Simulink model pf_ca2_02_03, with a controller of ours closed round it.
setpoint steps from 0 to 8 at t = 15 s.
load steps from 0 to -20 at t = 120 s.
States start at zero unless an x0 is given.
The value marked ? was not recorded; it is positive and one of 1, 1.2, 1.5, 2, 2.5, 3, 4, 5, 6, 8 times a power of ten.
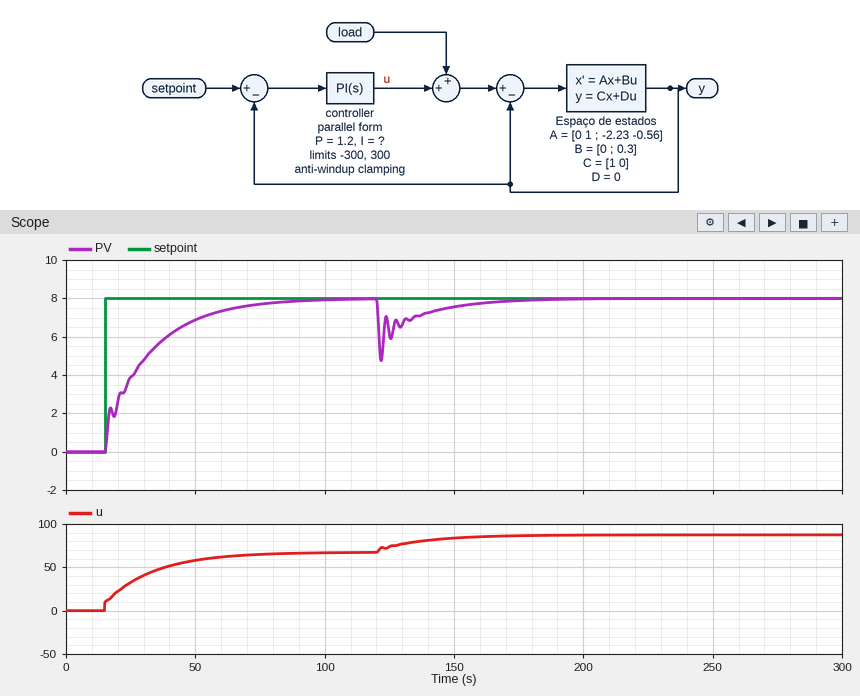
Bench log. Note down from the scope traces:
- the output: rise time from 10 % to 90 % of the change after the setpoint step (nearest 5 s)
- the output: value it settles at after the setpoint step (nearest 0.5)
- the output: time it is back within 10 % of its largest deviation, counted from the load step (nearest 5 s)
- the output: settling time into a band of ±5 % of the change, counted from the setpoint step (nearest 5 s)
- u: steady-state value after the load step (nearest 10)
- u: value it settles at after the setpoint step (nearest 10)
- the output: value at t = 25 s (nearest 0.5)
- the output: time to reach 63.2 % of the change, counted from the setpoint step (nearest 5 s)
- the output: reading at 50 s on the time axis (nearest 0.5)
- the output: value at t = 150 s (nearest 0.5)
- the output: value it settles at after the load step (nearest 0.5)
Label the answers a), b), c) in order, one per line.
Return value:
a) 40 s
b) 8.0
c) 35 s
d) 55 s
e) 90
f) 70
g) 4.0
h) 15 s
i) 7.0
j) 7.5
k) 8.0
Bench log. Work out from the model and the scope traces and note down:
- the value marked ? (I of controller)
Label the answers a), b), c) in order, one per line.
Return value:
a) 0.5
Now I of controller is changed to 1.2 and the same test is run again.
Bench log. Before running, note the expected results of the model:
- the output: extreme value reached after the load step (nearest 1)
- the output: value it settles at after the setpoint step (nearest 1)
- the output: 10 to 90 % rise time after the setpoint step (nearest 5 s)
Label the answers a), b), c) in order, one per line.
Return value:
a) 5
b) 8
c) 15 s
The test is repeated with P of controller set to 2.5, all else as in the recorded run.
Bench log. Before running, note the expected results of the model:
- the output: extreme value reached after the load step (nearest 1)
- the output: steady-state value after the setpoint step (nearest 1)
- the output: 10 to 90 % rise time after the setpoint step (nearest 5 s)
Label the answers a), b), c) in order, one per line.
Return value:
a) 5
b) 8
c) 45 s
